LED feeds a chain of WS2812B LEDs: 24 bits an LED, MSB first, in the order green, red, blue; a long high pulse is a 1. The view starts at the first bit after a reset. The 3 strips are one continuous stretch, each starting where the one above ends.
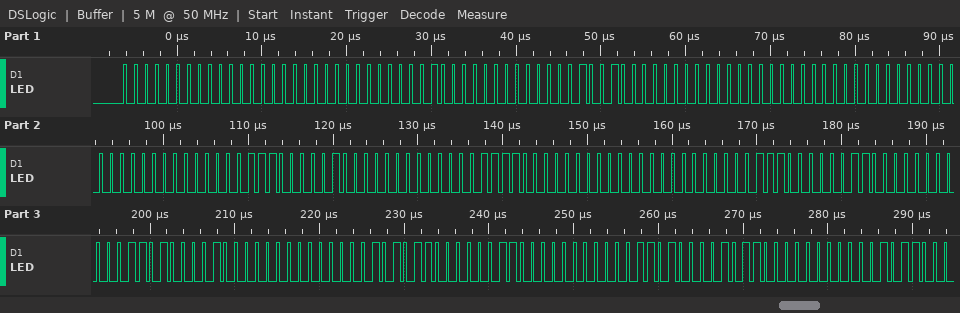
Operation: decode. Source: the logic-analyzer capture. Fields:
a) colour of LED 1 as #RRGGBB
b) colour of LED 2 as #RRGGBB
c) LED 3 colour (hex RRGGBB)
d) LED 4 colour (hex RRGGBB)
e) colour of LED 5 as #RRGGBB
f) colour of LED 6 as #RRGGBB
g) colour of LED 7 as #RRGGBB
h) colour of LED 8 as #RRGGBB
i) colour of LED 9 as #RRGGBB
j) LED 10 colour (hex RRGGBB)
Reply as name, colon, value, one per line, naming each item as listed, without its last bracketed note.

colour of LED 1 as #RRGGBB: #000000
colour of LED 2 as #RRGGBB: #000412
LED 3 colour: #000000
LED 4 colour: #000007
colour of LED 5 as #RRGGBB: #00041E
colour of LED 6 as #RRGGBB: #000007
colour of LED 7 as #RRGGBB: #00031A
colour of LED 8 as #RRGGBB: #00102B
colour of LED 9 as #RRGGBB: #00031A
LED 10 colour: #00162C
